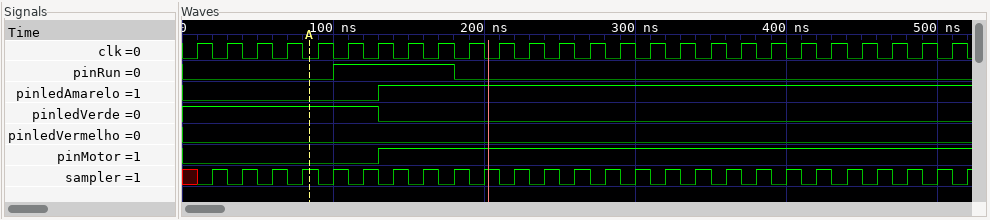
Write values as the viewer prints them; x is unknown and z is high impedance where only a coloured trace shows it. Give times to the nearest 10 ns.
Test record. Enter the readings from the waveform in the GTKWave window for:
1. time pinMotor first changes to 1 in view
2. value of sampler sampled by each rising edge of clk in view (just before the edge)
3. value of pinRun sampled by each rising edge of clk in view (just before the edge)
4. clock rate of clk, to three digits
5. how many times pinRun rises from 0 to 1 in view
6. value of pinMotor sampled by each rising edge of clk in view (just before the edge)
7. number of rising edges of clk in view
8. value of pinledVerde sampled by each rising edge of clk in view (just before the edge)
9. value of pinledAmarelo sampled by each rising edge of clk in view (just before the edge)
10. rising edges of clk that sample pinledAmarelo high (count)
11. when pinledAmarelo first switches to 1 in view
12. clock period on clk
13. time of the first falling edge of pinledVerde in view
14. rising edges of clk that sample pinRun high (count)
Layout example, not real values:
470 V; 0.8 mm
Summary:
130 ns; x 1 1 1 1 1 1 1 1 1 1 1 1 1 1 1 1 1 1 1 1 1 1 1 1 1; 0 0 0 0 0 1 1 1 1 0 0 0 0 0 0 0 0 0 0 0 0 0 0 0 0 0; 50.0 MHz; 1; 0 0 0 0 0 0 0 1 1 1 1 1 1 1 1 1 1 1 1 1 1 1 1 1 1 1; 26; 1 1 1 1 1 1 1 0 0 0 0 0 0 0 0 0 0 0 0 0 0 0 0 0 0 0; 0 0 0 0 0 0 0 1 1 1 1 1 1 1 1 1 1 1 1 1 1 1 1 1 1 1; 19; 130 ns; 20 ns; 130 ns; 4
